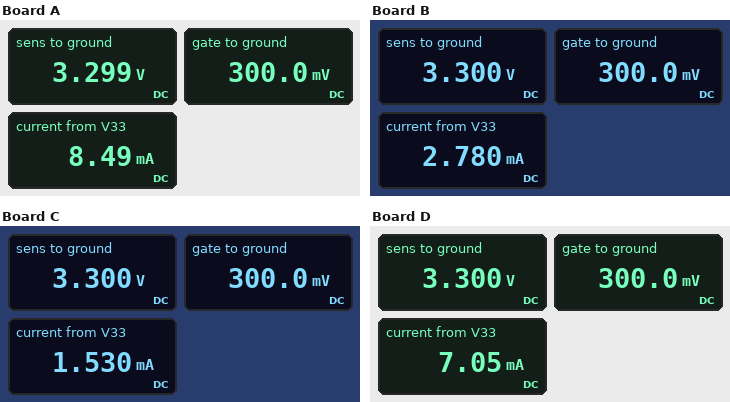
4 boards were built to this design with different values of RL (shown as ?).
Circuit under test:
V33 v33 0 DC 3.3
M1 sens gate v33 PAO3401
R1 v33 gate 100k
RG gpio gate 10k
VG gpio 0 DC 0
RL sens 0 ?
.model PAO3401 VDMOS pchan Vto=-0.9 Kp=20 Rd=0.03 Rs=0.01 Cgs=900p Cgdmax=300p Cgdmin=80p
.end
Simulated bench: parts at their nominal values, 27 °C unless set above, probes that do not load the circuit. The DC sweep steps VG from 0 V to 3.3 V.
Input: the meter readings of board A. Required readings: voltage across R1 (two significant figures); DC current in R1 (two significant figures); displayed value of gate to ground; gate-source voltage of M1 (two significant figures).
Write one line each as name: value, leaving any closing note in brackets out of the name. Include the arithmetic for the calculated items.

voltage across R1: 3.3 V - 300 mV = 3.0 V
DC current in R1: (3.3 V - 300 mV) / 100 kΩ = 30 µA
displayed value of gate to ground: 300.0 mV
gate-source voltage of M1: 300 mV - 3.3 V = -3.0 V
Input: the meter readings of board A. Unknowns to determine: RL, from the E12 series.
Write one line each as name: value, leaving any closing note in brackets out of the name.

RL, from the E12 series: 390 Ω
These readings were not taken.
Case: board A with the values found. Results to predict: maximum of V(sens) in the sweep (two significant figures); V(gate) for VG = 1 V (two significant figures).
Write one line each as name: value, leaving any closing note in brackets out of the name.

maximum of V(sens) in the sweep: 3.3 V
V(gate) for VG = 1 V: 1.2 V
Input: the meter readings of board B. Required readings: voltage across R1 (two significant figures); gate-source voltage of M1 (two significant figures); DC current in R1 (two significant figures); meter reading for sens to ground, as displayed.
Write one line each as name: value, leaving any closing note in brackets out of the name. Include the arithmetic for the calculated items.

voltage across R1: 3.3 V - 300 mV = 3.0 V
gate-source voltage of M1: 300 mV - 3.3 V = -3.0 V
DC current in R1: (3.3 V - 300 mV) / 100 kΩ = 30 µA
meter reading for sens to ground, as displayed: 3.300 V
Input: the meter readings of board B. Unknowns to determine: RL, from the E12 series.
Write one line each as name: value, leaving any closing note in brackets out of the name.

RL, from the E12 series: 1.2 kΩ
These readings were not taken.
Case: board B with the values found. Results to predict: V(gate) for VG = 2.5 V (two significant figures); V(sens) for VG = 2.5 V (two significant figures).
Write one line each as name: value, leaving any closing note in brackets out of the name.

V(gate) for VG = 2.5 V: 2.6 V
V(sens) for VG = 2.5 V: 3.2 V
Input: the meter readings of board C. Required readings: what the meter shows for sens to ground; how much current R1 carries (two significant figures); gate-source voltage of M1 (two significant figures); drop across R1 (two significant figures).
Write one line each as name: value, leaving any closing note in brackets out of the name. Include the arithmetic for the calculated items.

what the meter shows for sens to ground: 3.300 V
how much current R1 carries: (3.3 V - 300 mV) / 100 kΩ = 30 µA
gate-source voltage of M1: 300 mV - 3.3 V = -3.0 V
drop across R1: 3.3 V - 300 mV = 3.0 V
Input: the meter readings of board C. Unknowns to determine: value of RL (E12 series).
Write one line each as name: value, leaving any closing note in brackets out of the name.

value of RL: 2.2 kΩ
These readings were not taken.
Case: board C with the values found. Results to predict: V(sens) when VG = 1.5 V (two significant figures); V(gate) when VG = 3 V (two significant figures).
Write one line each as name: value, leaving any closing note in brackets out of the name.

V(sens) when VG = 1.5 V: 3.3 V
V(gate) when VG = 3 V: 3.0 V
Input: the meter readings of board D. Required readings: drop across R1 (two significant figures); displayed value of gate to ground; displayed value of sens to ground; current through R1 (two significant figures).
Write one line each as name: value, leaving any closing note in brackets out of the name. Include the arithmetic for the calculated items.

drop across R1: 3.3 V - 300 mV = 3.0 V
displayed value of gate to ground: 300.0 mV
displayed value of sens to ground: 3.300 V
current through R1: (3.3 V - 300 mV) / 100 kΩ = 30 µA
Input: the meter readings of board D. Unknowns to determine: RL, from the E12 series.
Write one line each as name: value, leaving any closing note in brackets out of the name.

RL, from the E12 series: 470 Ω
